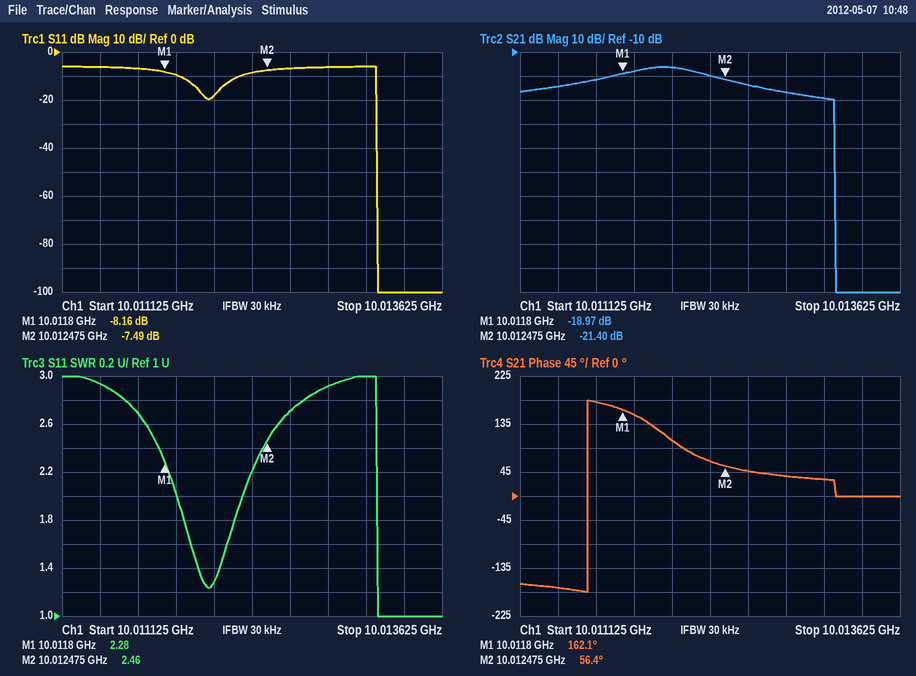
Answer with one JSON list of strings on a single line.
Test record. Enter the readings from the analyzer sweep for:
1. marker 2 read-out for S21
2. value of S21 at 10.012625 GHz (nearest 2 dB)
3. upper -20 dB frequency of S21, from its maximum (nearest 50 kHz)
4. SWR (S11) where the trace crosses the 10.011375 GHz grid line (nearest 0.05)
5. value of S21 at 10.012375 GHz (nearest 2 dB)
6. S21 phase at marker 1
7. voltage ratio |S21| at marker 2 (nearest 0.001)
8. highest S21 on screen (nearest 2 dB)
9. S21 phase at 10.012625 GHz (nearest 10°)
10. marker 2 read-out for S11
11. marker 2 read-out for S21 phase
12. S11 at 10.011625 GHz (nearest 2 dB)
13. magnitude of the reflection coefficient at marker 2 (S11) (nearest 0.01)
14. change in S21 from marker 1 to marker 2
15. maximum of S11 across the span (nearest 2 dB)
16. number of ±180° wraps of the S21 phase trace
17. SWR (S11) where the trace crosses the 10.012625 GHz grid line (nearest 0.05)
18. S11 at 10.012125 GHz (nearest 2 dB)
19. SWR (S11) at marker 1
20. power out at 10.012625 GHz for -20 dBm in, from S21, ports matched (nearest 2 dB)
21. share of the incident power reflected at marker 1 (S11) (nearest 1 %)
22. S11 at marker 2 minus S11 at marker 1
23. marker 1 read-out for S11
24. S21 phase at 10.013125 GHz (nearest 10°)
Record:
["-21.40 dB", "-24 dB", "10.01320 GHz", "2.95", "-20 dB", "162.1°", "0.085", "-16 dB", "50°", "-7.49 dB", "56.4°", "-6 dB", "0.42", "-2.43 dB", "-6 dB", "1", "2.70", "-18 dB", "2.28", "-44 dBm", "15 %", "0.67 dB", "-8.16 dB", "30°"]
